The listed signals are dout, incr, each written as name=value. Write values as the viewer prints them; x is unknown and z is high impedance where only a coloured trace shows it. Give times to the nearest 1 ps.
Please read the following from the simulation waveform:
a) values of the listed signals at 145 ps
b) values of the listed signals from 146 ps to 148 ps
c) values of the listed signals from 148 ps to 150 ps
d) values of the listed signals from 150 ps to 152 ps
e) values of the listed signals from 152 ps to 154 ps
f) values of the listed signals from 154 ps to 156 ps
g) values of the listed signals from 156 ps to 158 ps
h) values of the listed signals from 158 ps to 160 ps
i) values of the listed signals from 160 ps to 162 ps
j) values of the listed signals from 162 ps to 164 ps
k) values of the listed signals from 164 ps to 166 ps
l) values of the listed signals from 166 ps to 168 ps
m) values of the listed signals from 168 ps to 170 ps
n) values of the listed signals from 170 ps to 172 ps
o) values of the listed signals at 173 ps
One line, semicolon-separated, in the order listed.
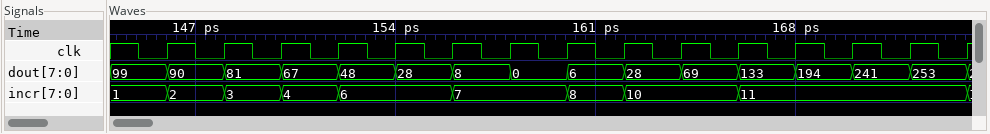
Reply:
dout=99, incr=1; dout=90, incr=2; dout=81, incr=3; dout=67, incr=4; dout=48, incr=6; dout=28, incr=6; dout=8, incr=7; dout=0, incr=7; dout=6, incr=8; dout=28, incr=10; dout=69, incr=10; dout=133, incr=11; dout=194, incr=11; dout=241, incr=11; dout=253, incr=11
